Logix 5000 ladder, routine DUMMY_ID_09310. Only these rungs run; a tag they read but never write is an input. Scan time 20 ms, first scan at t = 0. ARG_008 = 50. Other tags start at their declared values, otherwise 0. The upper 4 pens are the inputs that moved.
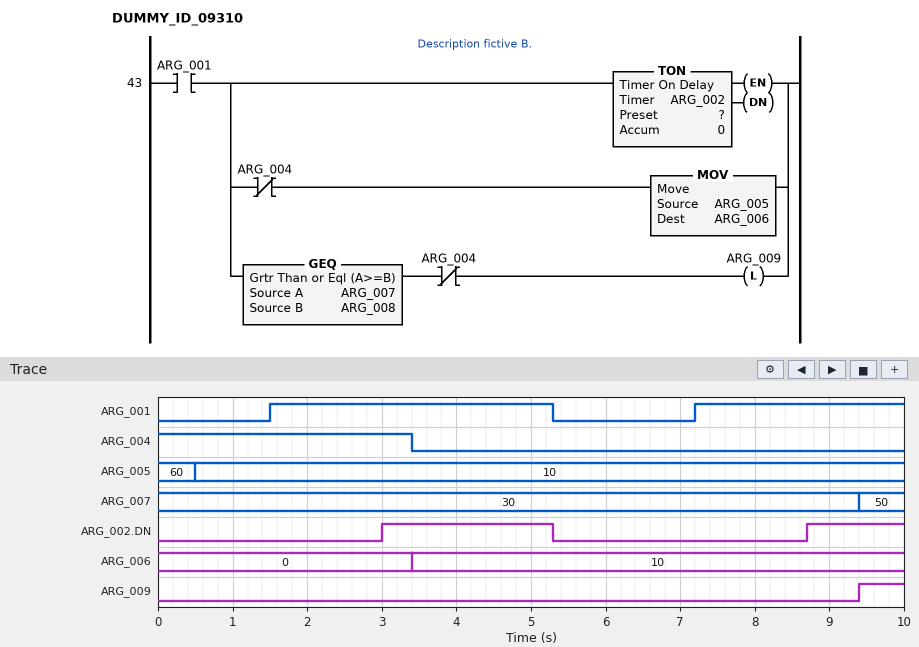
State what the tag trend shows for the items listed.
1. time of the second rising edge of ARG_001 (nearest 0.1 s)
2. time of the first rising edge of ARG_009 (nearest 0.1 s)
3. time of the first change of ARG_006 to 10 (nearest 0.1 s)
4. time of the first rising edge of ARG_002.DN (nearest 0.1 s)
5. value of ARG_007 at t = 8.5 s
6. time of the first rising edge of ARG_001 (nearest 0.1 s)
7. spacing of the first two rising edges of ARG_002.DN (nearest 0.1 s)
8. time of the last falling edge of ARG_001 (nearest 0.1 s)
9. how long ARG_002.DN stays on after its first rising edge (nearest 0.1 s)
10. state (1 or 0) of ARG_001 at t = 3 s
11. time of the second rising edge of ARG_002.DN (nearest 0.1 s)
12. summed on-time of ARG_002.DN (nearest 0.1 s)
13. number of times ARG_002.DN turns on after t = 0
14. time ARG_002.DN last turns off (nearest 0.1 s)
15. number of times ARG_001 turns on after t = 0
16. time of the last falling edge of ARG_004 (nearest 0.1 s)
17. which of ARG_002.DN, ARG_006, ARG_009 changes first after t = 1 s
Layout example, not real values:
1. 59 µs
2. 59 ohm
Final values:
1. 7.2 s
2. 9.4 s
3. 3.4 s
4. 3.0 s
5. 30
6. 1.5 s
7. 5.7 s
8. 5.3 s
9. 2.3 s
10. 1
11. 8.7 s
12. 3.6 s
13. 2
14. 5.3 s
15. 2
16. 3.4 s
17. ARG_002.DN
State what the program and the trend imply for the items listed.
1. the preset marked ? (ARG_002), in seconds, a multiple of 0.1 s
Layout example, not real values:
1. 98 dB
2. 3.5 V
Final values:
1. 1.5 s
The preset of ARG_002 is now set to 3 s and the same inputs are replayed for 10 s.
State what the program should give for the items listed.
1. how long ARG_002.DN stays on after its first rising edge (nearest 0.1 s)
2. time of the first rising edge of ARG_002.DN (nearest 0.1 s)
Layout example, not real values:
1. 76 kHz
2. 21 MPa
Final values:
1. 0.8 s
2. 4.5 s
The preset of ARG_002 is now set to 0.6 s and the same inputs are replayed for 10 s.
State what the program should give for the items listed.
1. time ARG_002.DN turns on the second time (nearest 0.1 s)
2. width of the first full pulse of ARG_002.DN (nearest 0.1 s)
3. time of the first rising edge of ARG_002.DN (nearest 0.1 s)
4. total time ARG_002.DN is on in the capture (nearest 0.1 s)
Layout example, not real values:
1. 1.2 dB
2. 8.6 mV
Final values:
1. 7.8 s
2. 3.2 s
3. 2.1 s
4. 5.4 s
